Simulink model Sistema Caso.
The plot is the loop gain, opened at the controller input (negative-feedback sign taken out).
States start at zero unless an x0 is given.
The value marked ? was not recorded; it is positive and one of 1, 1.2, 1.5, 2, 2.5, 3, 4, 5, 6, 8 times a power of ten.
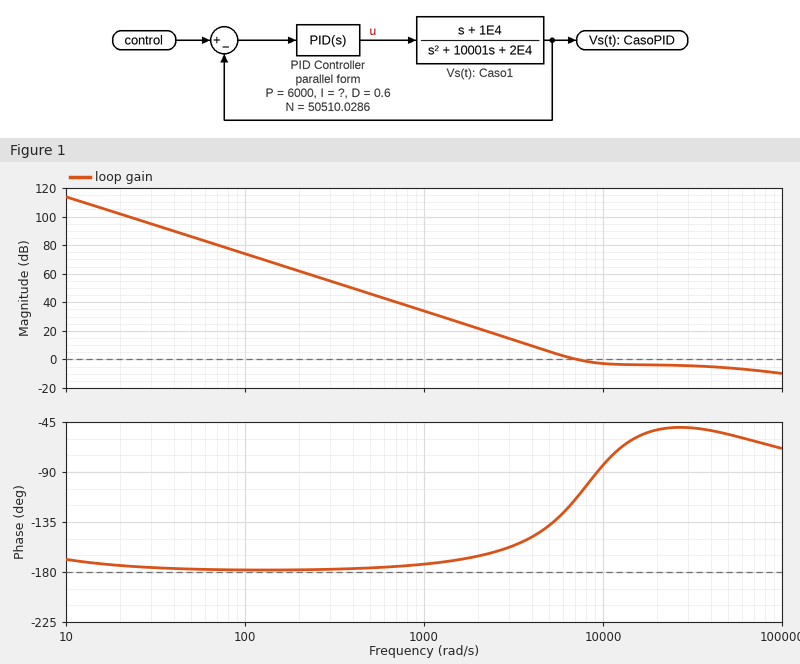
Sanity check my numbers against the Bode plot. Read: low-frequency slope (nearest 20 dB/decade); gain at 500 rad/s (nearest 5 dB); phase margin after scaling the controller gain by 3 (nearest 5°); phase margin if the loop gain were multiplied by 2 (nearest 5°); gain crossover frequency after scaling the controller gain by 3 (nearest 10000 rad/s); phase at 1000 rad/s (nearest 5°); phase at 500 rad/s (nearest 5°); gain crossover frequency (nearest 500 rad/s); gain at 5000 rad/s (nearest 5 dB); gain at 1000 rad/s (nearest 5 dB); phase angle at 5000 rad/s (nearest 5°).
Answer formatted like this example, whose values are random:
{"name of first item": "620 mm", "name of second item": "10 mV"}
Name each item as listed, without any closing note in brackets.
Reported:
{"low-frequency slope": "-40 dB/decade", "gain at 500 rad/s": "45 dB", "phase margin after scaling the controller gain by 3": "110°", "phase margin if the loop gain were multiplied by 2": "125°", "gain crossover frequency after scaling the controller gain by 3": "100000 rad/s", "phase at 1000 rad/s": "-175°", "phase at 500 rad/s": "-175°", "gain crossover frequency": "7000 rad/s", "gain at 5000 rad/s": "5 dB", "gain at 1000 rad/s": "35 dB", "phase angle at 5000 rad/s": "-140°"}
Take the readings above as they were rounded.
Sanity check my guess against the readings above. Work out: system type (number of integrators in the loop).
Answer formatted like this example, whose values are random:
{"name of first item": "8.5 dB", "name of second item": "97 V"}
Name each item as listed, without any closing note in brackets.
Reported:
{"system type": "2"}
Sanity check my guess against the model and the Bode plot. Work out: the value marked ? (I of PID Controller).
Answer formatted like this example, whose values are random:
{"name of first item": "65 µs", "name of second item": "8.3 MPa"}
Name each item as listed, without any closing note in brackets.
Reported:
{"the value marked ?": "5e+07"}
